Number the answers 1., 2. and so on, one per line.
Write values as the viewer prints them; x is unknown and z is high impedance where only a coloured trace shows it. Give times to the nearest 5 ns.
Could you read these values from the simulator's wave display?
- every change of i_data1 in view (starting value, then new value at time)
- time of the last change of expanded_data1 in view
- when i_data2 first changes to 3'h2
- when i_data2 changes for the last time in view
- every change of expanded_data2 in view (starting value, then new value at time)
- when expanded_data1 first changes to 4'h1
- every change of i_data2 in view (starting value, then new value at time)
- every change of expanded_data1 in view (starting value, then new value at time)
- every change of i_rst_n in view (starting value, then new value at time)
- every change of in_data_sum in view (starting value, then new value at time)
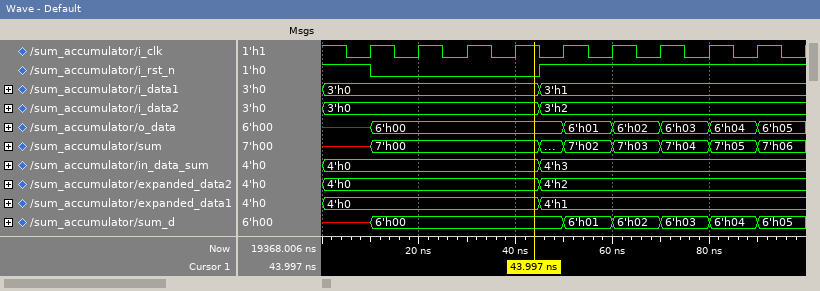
1. 3'h0, 3'h1 at 45 ns
2. 45 ns
3. 45 ns
4. 45 ns
5. 4'h0, 4'h2 at 45 ns
6. 45 ns
7. 3'h0, 3'h2 at 45 ns
8. 4'h0, 4'h1 at 45 ns
9. 1, 0 at 10 ns, 1 at 45 ns
10. 4'h0, 4'h3 at 45 ns
